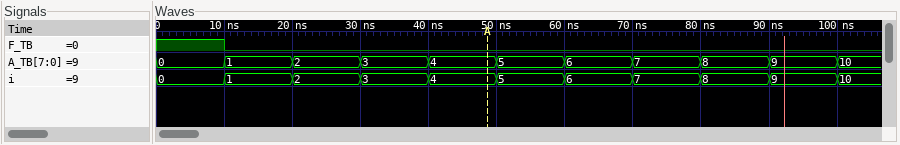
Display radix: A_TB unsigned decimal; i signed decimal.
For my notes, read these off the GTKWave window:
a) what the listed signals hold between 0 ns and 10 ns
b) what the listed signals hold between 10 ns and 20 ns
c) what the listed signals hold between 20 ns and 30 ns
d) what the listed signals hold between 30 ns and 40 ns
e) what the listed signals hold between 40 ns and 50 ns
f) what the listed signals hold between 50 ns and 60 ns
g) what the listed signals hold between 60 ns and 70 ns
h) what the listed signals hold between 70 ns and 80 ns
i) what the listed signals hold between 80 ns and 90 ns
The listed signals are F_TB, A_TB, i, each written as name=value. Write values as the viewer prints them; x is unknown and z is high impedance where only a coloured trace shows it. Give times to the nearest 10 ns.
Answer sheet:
F_TB=1, A_TB=0, i=0
F_TB=0, A_TB=1, i=1
F_TB=0, A_TB=2, i=2
F_TB=0, A_TB=3, i=3
F_TB=0, A_TB=4, i=4
F_TB=0, A_TB=5, i=5
F_TB=0, A_TB=6, i=6
F_TB=0, A_TB=7, i=7
F_TB=0, A_TB=8, i=8
